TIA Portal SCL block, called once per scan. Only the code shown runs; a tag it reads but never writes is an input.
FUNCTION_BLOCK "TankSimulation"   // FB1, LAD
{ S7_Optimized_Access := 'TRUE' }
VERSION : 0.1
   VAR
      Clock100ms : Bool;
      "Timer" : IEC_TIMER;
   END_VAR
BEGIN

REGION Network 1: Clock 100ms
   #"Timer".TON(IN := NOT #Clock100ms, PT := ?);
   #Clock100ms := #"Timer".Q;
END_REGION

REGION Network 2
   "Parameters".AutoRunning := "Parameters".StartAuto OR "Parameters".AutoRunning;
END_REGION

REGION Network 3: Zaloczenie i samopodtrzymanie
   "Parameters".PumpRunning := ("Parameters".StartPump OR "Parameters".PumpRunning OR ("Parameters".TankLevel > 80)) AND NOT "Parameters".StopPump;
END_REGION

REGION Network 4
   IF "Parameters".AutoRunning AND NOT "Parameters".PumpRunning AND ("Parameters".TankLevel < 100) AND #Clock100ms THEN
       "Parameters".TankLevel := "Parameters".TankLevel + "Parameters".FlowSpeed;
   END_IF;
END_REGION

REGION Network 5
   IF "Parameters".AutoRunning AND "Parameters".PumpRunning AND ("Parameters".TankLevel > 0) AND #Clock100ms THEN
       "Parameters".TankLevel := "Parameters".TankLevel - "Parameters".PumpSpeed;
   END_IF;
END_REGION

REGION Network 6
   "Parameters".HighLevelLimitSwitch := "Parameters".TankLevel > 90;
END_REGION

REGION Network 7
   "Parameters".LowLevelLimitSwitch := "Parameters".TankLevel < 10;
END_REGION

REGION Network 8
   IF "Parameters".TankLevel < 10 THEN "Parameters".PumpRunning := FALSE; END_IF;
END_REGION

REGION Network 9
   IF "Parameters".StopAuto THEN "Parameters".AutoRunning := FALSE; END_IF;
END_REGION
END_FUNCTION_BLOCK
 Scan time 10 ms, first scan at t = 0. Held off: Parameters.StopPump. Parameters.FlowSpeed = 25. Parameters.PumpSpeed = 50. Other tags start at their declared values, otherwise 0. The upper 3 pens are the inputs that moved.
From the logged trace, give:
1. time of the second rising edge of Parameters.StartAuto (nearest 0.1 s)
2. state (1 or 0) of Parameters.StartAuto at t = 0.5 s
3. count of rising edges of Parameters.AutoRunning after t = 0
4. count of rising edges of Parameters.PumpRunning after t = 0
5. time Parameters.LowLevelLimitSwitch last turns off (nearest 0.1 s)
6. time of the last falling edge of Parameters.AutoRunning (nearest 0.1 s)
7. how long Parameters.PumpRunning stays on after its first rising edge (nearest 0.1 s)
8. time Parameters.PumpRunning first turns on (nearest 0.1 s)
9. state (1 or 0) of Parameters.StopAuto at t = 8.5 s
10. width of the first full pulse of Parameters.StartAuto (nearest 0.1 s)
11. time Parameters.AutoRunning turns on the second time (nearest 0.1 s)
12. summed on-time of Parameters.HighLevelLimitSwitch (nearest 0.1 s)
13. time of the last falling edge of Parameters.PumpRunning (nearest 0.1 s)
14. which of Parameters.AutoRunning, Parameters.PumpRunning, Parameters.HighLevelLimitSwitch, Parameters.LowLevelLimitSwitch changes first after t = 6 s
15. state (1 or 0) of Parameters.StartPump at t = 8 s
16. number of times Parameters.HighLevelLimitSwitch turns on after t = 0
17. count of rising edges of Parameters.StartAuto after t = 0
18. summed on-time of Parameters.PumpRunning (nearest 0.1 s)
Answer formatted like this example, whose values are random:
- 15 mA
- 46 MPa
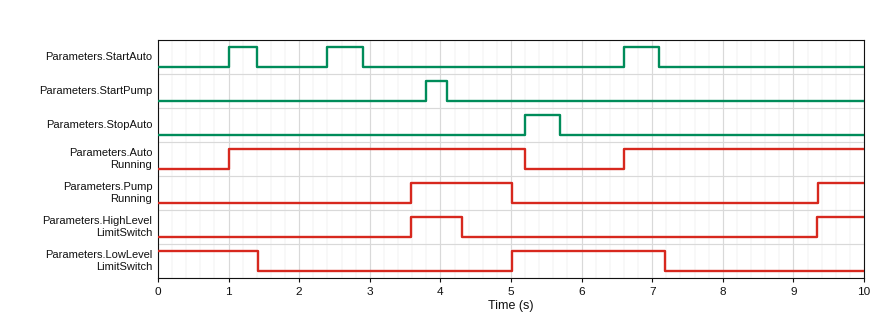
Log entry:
- 2.4 s
- 0
- 2
- 2
- 7.2 s
- 5.2 s
- 1.4 s
- 3.6 s
- 0
- 0.4 s
- 6.6 s
- 1.4 s
- 5.0 s
- Parameters.AutoRunning
- 0
- 2
- 3
- 2.1 s
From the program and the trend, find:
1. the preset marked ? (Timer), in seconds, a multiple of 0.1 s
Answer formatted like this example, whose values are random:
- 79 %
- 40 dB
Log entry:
- 0.7 s
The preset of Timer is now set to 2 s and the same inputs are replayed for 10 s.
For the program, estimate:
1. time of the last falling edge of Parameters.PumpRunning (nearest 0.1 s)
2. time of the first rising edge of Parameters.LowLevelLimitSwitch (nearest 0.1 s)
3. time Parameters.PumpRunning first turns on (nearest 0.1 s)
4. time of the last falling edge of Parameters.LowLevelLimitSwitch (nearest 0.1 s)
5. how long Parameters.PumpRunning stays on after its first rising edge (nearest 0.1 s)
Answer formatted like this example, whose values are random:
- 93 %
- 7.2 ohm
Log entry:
- 4.0 s
- 4.0 s
- 3.8 s
- 2.0 s
- 0.2 s
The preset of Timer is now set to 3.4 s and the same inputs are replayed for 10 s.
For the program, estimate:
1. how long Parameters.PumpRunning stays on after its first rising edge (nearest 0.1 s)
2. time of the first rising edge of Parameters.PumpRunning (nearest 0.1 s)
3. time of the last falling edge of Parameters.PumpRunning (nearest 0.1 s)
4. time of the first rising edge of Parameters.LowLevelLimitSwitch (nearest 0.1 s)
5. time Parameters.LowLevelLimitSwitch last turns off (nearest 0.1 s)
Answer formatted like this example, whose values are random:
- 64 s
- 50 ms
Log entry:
- 3.0 s
- 3.8 s
- 6.8 s
- 6.8 s
- 3.4 s
